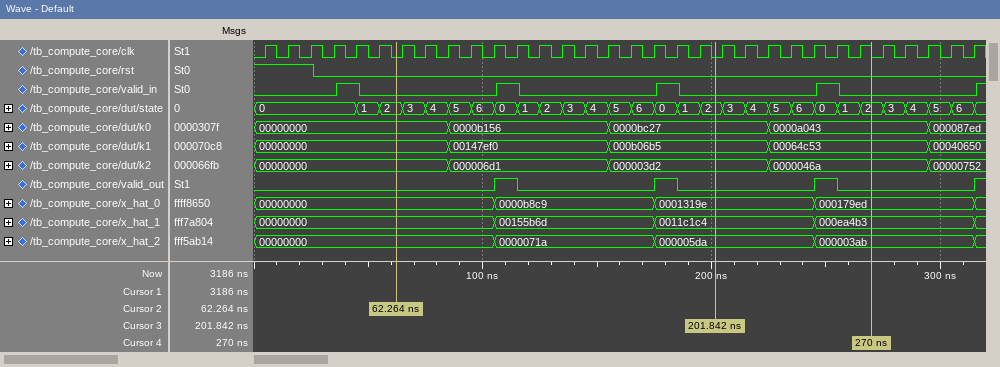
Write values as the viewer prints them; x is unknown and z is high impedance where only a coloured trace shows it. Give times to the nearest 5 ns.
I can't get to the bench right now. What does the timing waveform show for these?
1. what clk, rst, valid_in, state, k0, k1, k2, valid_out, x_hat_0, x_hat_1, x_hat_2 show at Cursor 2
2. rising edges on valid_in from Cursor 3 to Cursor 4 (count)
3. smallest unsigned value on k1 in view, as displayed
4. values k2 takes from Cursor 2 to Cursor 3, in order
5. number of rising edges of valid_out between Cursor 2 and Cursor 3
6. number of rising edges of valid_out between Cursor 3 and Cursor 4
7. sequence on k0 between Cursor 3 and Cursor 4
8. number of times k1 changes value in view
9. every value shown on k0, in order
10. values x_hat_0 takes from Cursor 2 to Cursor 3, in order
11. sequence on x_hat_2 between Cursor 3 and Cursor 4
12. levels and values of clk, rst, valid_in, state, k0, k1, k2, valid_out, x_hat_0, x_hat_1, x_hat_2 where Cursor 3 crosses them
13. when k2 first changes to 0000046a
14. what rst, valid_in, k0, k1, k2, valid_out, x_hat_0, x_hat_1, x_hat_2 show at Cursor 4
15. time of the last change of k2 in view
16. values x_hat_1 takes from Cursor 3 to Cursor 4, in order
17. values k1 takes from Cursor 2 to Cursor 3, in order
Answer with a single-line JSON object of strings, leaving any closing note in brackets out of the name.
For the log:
{"what clk, rst, valid_in, state, k0, k1, k2, valid_out, x_hat_0, x_hat_1, x_hat_2 show at Cursor 2": "clk=0, rst=0, valid_in=0, state=2, k0=00000000, k1=00000000, k2=00000000, valid_out=0, x_hat_0=00000000, x_hat_1=00000000, x_hat_2=00000000", "rising edges on valid_in from Cursor 3 to Cursor 4": "1", "smallest unsigned value on k1 in view, as displayed": "00000000", "values k2 takes from Cursor 2 to Cursor 3, in order": "00000000, 000006d1, 000003d2", "number of rising edges of valid_out between Cursor 2 and Cursor 3": "2", "number of rising edges of valid_out between Cursor 3 and Cursor 4": "1", "sequence on k0 between Cursor 3 and Cursor 4": "0000bc27, 0000a043", "number of times k1 changes value in view": "4", "every value shown on k0, in order": "00000000, 0000b156, 0000bc27, 0000a043, 000087ed", "values x_hat_0 takes from Cursor 2 to Cursor 3, in order": "00000000, 0000b8c9, 0001319e", "sequence on x_hat_2 between Cursor 3 and Cursor 4": "000005da, 000003ab", "levels and values of clk, rst, valid_in, state, k0, k1, k2, valid_out, x_hat_0, x_hat_1, x_hat_2 where Cursor 3 crosses them": "clk=0, rst=0, valid_in=0, state=2, k0=0000bc27, k1=000b06b5, k2=000003d2, valid_out=0, x_hat_0=0001319e, x_hat_1=0011c1c4, x_hat_2=000005da", "when k2 first changes to 0000046a": "225 ns", "what rst, valid_in, k0, k1, k2, valid_out, x_hat_0, x_hat_1, x_hat_2 show at Cursor 4": "rst=0, valid_in=0, k0=0000a043, k1=00064c53, k2=0000046a, valid_out=0, x_hat_0=000179ed, x_hat_1=000ea4b3, x_hat_2=000003ab", "time of the last change of k2 in view": "295 ns", "values x_hat_1 takes from Cursor 3 to Cursor 4, in order": "0011c1c4, 000ea4b3", "values k1 takes from Cursor 2 to Cursor 3, in order": "00000000, 00147ef0, 000b06b5"}
